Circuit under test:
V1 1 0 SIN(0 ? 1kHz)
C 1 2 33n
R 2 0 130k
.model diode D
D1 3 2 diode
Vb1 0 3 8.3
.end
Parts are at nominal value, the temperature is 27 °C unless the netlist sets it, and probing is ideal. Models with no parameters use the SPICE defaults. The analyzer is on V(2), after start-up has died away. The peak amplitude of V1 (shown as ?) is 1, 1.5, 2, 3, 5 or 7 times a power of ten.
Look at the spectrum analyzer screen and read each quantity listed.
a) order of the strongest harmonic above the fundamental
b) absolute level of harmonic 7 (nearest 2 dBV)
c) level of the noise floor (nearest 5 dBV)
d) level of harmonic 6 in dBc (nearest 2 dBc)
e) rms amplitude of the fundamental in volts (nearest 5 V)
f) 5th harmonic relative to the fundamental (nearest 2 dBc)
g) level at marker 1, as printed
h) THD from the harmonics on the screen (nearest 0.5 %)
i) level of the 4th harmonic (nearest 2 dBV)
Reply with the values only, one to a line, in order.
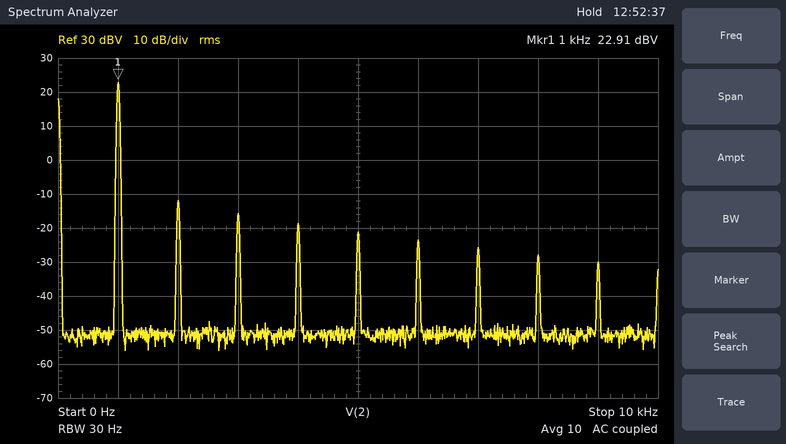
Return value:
2
-26 dBV
-50 dBV
-46 dBc
15 V
-44 dBc
22.91 dBV
2.5 %
-18 dBV
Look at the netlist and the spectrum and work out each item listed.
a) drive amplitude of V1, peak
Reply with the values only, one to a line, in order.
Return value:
20 V
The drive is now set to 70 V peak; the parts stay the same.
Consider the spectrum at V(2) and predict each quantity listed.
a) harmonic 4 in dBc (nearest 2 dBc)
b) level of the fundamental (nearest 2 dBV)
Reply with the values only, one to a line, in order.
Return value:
-38 dBc
34 dBV
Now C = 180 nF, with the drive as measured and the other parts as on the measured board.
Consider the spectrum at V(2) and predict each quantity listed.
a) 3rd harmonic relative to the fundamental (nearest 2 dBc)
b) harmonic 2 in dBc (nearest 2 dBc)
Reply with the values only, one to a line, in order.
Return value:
-52 dBc
-48 dBc
